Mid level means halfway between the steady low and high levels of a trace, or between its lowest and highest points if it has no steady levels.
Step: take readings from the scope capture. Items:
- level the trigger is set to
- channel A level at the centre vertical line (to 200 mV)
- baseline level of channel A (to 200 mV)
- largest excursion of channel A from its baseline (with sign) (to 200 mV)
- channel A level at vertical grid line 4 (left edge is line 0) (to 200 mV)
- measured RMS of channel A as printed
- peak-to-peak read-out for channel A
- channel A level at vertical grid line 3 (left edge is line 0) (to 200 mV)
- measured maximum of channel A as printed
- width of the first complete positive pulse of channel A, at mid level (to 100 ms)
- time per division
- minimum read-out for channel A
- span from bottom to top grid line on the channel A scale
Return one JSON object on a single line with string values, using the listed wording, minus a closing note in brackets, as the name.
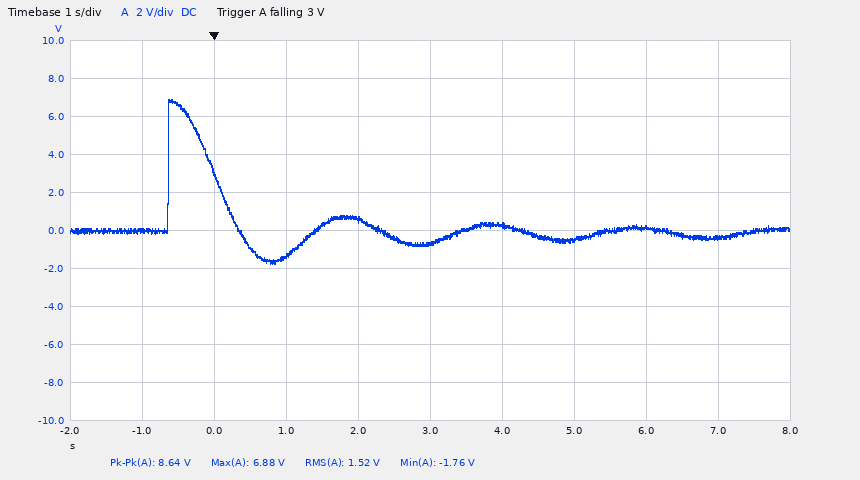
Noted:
{"level the trigger is set to": "3 V", "channel A level at the centre vertical line": "-600 mV", "baseline level of channel A": "0.0 V", "largest excursion of channel A from its baseline (with sign)": "+6.8 V", "channel A level at vertical grid line 4 (left edge is line 0)": "600 mV", "measured RMS of channel A as printed": "1.52 V", "peak-to-peak read-out for channel A": "8.64 V", "channel A level at vertical grid line 3 (left edge is line 0)": "-1.4 V", "measured maximum of channel A as printed": "6.88 V", "width of the first complete positive pulse of channel A, at mid level": "700 ms", "time per division": "1 s", "minimum read-out for channel A": "-1.76 V", "span from bottom to top grid line on the channel A scale": "20 V"}
